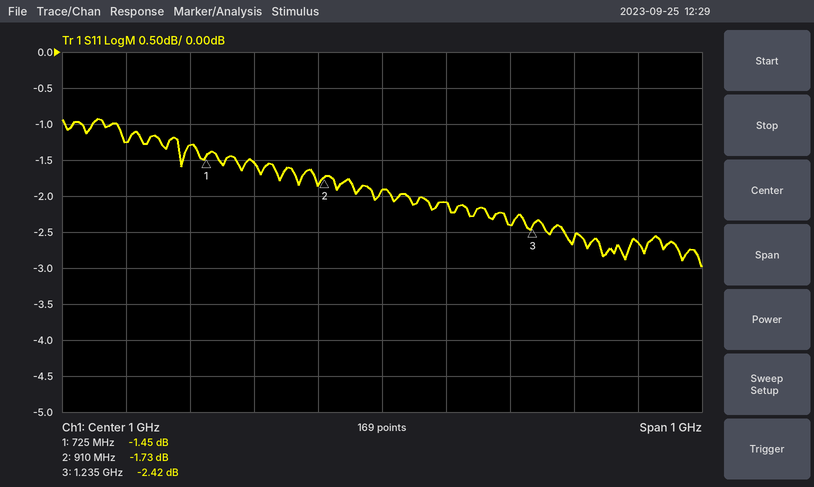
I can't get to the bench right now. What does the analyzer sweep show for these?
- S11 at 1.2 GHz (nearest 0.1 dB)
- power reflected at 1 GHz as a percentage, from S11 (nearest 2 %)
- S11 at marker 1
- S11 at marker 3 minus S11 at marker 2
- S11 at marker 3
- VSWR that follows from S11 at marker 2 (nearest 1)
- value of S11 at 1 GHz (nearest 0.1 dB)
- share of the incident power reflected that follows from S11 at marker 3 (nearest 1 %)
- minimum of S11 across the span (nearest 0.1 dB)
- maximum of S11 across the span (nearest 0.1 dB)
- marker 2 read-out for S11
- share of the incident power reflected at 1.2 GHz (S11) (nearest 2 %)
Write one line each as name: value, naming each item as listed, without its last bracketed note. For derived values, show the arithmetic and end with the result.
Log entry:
S11 at 1.2 GHz: -2.4 dB
power reflected at 1 GHz as a percentage, from S11: 10^(-1.9/10) ≈ 64.6 %, so 64 % to the nearest 2 %
S11 at marker 1: -1.45 dB
S11 at marker 3 minus S11 at marker 2: -2.42 − (-1.73) = -0.69 dB
S11 at marker 3: -2.42 dB
VSWR that follows from S11 at marker 2: (1 + 0.8194)/(1 − 0.8194) ≈ 10
value of S11 at 1 GHz: -1.9 dB
share of the incident power reflected that follows from S11 at marker 3: 10^(-2.42/10) ≈ 57 %
minimum of S11 across the span: -3.0 dB
maximum of S11 across the span: -0.9 dB
marker 2 read-out for S11: -1.73 dB
share of the incident power reflected at 1.2 GHz (S11): 10^(-2.4/10) ≈ 58 %
